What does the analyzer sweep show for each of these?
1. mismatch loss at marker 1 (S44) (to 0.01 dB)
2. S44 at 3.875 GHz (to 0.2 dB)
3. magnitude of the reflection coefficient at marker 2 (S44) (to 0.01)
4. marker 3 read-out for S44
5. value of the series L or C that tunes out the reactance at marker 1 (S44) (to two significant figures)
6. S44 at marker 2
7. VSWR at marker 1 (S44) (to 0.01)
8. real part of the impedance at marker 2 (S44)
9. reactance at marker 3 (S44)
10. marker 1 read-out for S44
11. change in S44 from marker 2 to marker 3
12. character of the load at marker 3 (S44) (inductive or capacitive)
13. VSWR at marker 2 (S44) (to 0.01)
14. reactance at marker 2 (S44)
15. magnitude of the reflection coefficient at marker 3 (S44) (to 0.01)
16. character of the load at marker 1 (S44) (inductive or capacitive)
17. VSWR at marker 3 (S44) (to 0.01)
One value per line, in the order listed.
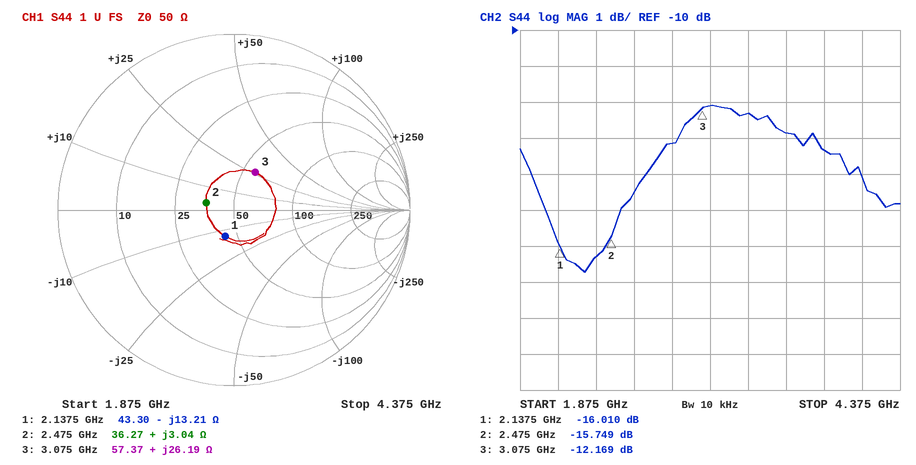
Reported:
0.11 dB
-13.4 dB
0.16
-12.169 dB
980 pH
-15.749 dB
1.37
36.27 Ω
+26.19 Ω
-16.010 dB
3.580 dB
inductive
1.39
+3.04 Ω
0.25
capacitive
1.65
